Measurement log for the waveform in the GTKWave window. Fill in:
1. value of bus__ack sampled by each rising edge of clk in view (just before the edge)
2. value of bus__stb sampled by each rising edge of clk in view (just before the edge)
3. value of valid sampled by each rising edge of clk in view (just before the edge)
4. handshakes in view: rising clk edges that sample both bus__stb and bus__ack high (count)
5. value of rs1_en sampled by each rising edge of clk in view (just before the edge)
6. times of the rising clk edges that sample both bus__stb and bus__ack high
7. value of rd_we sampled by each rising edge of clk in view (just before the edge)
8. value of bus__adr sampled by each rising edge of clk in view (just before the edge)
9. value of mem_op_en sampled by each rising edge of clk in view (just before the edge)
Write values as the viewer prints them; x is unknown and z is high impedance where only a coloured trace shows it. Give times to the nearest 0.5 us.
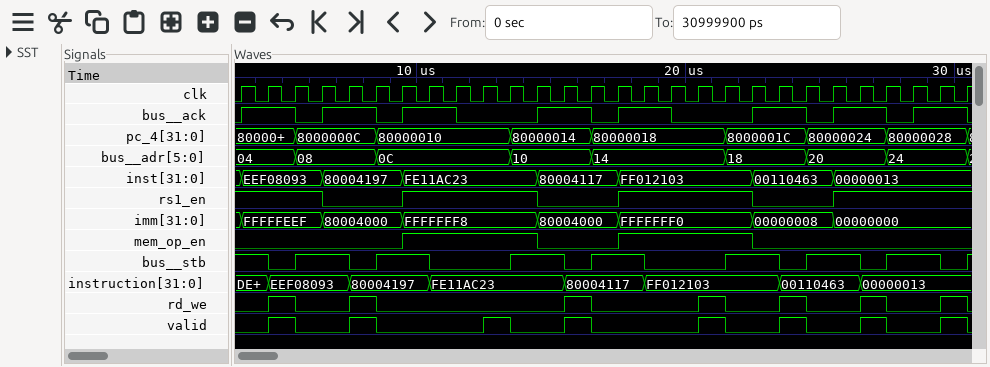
0 1 1 0 1 1 0 1 1 0 0 0 1 1 0 1 1 0 0 0 1 1 0 1 1 0 1 1
1 1 0 1 1 0 1 1 0 0 0 1 1 0 1 1 0 0 0 1 1 0 1 1 0 1 1 0
0 0 1 0 0 1 0 0 0 0 1 0 0 1 0 0 0 0 1 0 0 1 0 0 1 0 0 1
8
1 1 1 1 0 0 0 1 1 1 1 1 0 0 0 1 1 1 1 1 0 0 0 1 1 1 1 1
4.5 us, 7.5 us, 10.5 us, 15.5 us, 18.5 us, 23.5 us, 26.5 us, 29.5 us
0 0 1 0 0 1 0 0 0 0 0 0 0 1 0 0 0 0 1 0 0 1 0 0 1 0 0 1
04, 04, 04, 08, 08, 08, 0C, 0C, 0C, 0C, 0C, 10, 10, 10, 14, 14, 14, 14, 14, 18, 18, 18, 20, 20, 20, 24, 24, 24
0 0 0 0 0 0 0 1 1 1 1 1 0 0 0 1 1 1 1 1 0 0 0 0 0 0 0 0
